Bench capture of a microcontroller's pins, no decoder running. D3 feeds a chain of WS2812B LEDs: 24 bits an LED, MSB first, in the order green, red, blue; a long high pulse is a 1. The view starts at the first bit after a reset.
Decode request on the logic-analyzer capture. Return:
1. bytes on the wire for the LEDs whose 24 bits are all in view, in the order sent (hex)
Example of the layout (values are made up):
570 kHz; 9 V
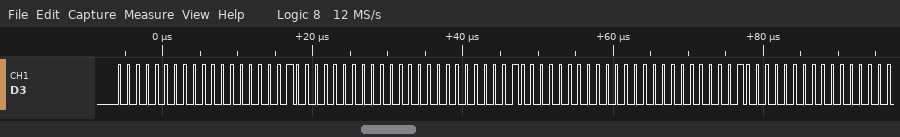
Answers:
00 00 20 00 00 20 00 00 20
